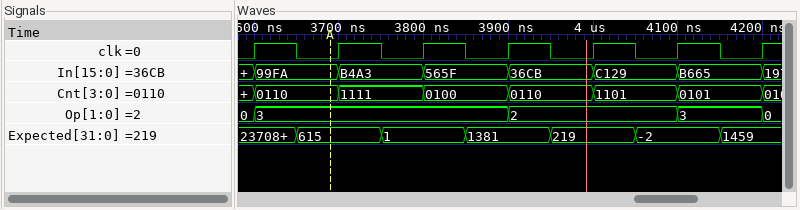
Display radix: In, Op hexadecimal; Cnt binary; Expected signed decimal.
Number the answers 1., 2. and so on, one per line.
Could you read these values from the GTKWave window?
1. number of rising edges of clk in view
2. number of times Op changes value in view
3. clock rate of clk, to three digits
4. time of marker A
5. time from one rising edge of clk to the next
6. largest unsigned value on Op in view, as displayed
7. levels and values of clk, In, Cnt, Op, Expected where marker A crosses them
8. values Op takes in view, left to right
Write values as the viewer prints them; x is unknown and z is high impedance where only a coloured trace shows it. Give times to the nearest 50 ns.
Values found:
1. 7
2. 4
3. 10.0 MHz
4. 3700 ns
5. 100 ns
6. 3
7. clk=0, In=99FA, Cnt=0110, Op=3, Expected=615
8. 0, 3, 2, 3, 0
